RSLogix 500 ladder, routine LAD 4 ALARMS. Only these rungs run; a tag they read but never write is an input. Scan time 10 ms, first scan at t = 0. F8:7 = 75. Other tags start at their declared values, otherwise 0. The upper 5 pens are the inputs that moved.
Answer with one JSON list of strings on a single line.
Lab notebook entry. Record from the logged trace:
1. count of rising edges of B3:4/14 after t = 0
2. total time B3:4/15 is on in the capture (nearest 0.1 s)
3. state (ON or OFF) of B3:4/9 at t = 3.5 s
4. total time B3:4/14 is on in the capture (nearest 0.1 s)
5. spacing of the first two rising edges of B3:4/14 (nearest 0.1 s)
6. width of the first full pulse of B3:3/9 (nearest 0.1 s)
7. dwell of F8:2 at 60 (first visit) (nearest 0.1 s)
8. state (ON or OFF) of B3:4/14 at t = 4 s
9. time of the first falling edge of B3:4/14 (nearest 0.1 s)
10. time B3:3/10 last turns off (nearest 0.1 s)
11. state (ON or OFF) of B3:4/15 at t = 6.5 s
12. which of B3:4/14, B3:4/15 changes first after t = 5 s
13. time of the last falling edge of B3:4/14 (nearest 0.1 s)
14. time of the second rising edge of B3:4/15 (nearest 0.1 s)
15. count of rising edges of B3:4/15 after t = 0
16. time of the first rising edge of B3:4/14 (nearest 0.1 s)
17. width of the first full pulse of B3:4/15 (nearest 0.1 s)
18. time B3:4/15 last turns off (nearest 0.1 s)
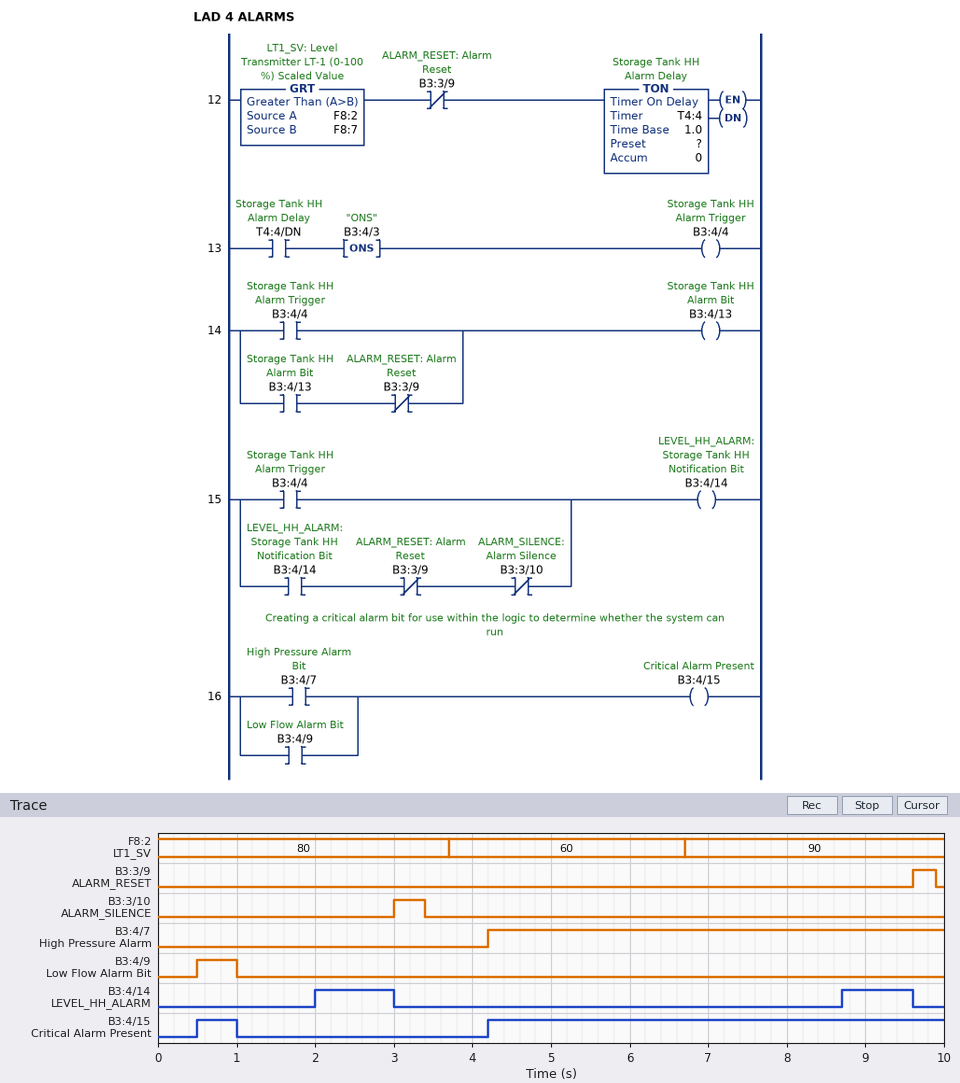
["2", "6.3 s", "OFF", "1.9 s", "6.7 s", "0.3 s", "3.0 s", "OFF", "3.0 s", "3.4 s", "ON", "B3:4/14", "9.6 s", "4.2 s", "2", "2.0 s", "0.5 s", "1.0 s"]
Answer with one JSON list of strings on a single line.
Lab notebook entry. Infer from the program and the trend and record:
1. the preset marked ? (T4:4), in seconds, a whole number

["2 s"]
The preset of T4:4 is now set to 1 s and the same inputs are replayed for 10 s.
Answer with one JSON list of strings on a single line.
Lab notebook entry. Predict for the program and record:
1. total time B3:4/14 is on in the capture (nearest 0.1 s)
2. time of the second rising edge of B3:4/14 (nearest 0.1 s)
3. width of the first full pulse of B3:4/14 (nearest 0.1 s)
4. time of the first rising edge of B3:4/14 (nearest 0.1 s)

["3.9 s", "7.7 s", "2.0 s", "1.0 s"]
